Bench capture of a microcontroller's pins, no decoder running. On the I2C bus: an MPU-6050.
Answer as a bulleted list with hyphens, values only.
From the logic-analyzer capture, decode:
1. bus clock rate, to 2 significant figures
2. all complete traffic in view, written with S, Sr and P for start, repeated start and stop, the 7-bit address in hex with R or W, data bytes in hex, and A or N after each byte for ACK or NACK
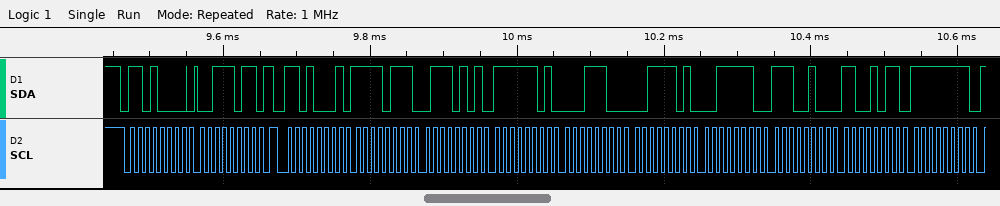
- 100 kHz
- S 68W A 3B A Sr 68R A F7 A 75 A FD A 1C A 3D A 3E A E4 A CB A FF A
